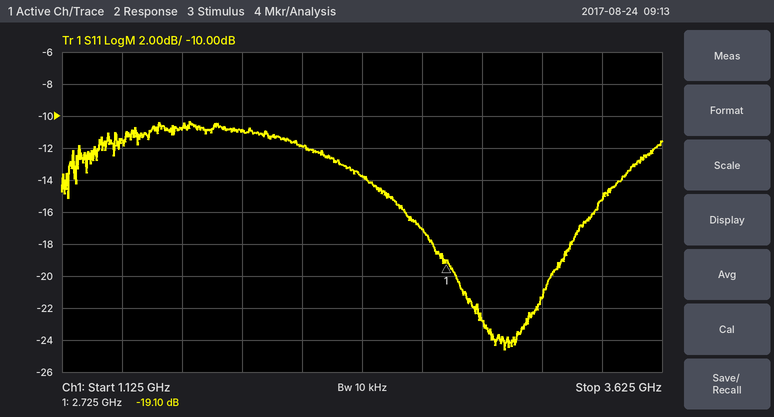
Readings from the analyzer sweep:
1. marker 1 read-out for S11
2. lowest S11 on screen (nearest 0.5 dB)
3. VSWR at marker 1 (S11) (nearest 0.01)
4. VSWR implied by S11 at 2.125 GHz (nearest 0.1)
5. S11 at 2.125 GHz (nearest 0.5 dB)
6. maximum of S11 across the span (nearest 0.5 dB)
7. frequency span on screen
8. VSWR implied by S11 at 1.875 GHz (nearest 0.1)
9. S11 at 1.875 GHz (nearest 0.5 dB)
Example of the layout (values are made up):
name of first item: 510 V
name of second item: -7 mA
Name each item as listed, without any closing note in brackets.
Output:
marker 1 read-out for S11: -19.10 dB
lowest S11 on screen: -24.5 dB
VSWR at marker 1 (S11): 1.25
VSWR implied by S11 at 2.125 GHz: 1.7
S11 at 2.125 GHz: -12.0 dB
maximum of S11 across the span: -10.5 dB
frequency span on screen: 2.5 GHz
VSWR implied by S11 at 1.875 GHz: 1.8
S11 at 1.875 GHz: -11.0 dB
